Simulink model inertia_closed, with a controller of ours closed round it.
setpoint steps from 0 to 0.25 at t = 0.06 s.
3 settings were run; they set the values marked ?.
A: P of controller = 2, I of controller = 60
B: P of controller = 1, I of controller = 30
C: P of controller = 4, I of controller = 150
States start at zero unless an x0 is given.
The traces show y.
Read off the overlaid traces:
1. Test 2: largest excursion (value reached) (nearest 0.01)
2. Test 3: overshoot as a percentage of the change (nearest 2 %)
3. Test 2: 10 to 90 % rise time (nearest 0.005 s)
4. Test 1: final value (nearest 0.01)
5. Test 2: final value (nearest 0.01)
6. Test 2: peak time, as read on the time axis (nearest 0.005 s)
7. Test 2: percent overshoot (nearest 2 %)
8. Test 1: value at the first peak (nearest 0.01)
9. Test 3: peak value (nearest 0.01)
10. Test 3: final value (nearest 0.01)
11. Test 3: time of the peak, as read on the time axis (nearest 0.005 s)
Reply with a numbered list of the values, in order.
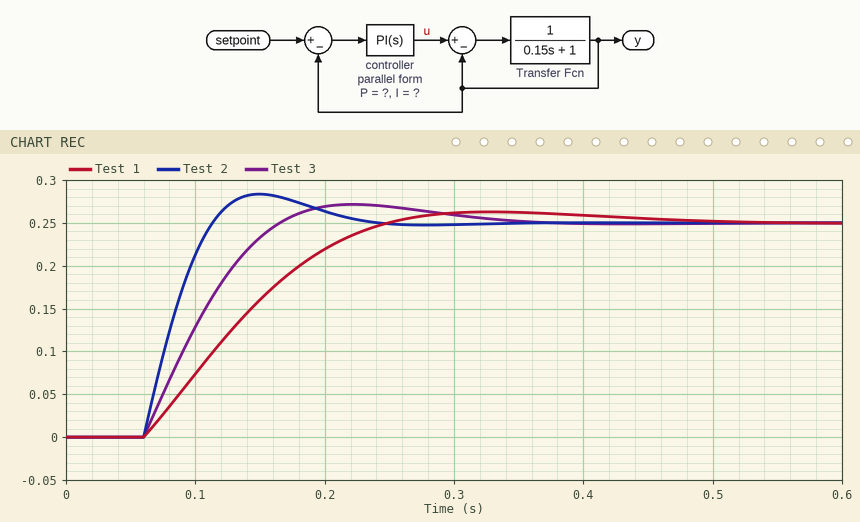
1. 0.28
2. 8 %
3. 0.040 s
4. 0.25
5. 0.25
6. 0.150 s
7. 14 %
8. 0.26
9. 0.27
10. 0.25
11. 0.220 s
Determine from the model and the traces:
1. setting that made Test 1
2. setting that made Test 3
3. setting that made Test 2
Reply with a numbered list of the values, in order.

1. B
2. A
3. C
